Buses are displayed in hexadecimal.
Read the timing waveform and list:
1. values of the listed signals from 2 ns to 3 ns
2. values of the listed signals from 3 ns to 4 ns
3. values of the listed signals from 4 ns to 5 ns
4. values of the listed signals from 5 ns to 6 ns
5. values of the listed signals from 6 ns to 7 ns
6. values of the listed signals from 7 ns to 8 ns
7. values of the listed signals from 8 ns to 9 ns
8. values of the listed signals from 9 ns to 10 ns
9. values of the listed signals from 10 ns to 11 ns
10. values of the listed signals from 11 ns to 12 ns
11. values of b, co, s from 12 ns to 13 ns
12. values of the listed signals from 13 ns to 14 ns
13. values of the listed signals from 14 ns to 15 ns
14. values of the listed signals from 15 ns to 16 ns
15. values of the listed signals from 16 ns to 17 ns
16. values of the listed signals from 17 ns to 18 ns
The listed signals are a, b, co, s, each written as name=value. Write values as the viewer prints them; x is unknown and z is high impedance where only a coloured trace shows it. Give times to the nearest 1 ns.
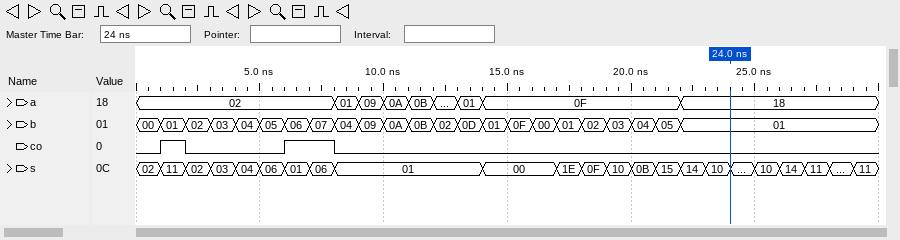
a=02, b=02, co=0, s=02
a=02, b=03, co=0, s=03
a=02, b=04, co=0, s=04
a=02, b=05, co=0, s=06
a=02, b=06, co=1, s=01
a=02, b=07, co=1, s=06
a=01, b=04, co=0, s=01
a=09, b=09, co=0, s=01
a=0A, b=0A, co=0, s=01
a=0B, b=0B, co=0, s=01
b=02, co=0, s=01
a=01, b=0D, co=0, s=01
a=0F, b=01, co=0, s=00
a=0F, b=0F, co=0, s=00
a=0F, b=00, co=0, s=00
a=0F, b=01, co=0, s=1E
